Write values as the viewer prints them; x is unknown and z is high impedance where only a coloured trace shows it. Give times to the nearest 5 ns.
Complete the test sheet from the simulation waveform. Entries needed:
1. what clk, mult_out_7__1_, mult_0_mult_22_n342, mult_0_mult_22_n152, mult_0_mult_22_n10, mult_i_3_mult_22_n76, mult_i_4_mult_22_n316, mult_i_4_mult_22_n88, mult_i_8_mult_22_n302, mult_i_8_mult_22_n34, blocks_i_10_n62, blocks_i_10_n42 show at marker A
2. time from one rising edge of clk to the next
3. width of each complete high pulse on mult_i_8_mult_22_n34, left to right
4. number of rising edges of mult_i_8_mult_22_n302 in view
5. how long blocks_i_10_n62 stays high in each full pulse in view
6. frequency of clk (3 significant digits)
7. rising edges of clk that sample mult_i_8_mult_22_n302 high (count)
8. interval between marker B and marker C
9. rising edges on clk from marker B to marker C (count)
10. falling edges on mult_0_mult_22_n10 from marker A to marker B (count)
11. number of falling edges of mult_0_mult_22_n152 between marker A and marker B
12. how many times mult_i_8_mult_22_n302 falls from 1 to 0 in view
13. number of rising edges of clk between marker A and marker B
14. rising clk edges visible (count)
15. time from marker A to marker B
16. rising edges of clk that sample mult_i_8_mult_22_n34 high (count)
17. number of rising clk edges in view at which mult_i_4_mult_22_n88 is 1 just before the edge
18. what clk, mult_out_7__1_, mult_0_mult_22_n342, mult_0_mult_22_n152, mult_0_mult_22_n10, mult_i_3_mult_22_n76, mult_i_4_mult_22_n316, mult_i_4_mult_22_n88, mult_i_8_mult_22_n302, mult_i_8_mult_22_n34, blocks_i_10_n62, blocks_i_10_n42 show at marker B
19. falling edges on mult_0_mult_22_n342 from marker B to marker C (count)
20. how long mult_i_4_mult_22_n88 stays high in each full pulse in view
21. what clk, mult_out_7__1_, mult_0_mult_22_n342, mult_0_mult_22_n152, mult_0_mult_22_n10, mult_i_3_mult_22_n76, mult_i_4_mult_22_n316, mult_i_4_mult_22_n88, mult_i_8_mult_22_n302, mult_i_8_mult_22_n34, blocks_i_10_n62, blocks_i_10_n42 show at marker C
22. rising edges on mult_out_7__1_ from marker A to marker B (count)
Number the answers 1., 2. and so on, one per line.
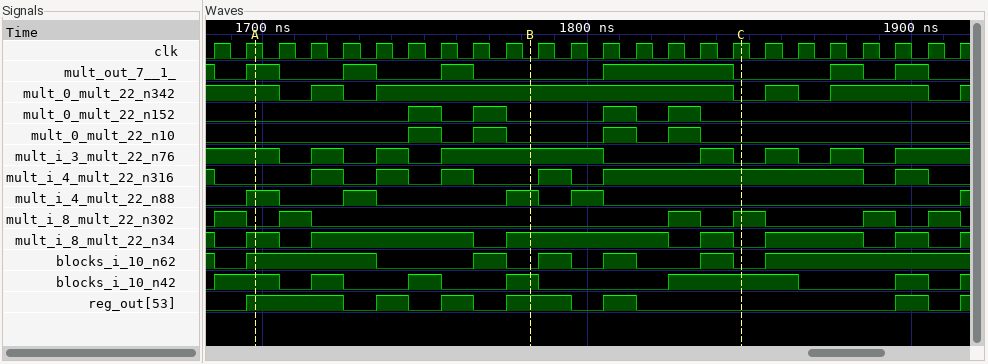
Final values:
1. clk=1, mult_out_7__1_=1, mult_0_mult_22_n342=1, mult_0_mult_22_n152=0, mult_0_mult_22_n10=0, mult_i_3_mult_22_n76=1, mult_i_4_mult_22_n316=0, mult_i_4_mult_22_n88=1, mult_i_8_mult_22_n302=0, mult_i_8_mult_22_n34=1, blocks_i_10_n62=1, blocks_i_10_n42=1
2. 10 ns
3. 10 ns, 50 ns, 50 ns, 10 ns, 30 ns, 10 ns
4. 6
5. 40 ns, 10 ns, 10 ns, 10 ns, 10 ns
6. 100 MHz
7. 6
8. 65 ns
9. 7
10. 2
11. 2
12. 6
13. 8
14. 24
15. 85 ns
16. 17
17. 4
18. clk=0, mult_out_7__1_=0, mult_0_mult_22_n342=1, mult_0_mult_22_n152=0, mult_0_mult_22_n10=0, mult_i_3_mult_22_n76=1, mult_i_4_mult_22_n316=0, mult_i_4_mult_22_n88=1, mult_i_8_mult_22_n302=0, mult_i_8_mult_22_n34=1, blocks_i_10_n62=0, blocks_i_10_n42=1
19. 1
20. 10 ns, 10 ns, 10 ns, 10 ns
21. clk=1, mult_out_7__1_=0, mult_0_mult_22_n342=0, mult_0_mult_22_n152=0, mult_0_mult_22_n10=0, mult_i_3_mult_22_n76=0, mult_i_4_mult_22_n316=1, mult_i_4_mult_22_n88=0, mult_i_8_mult_22_n302=1, mult_i_8_mult_22_n34=0, blocks_i_10_n62=0, blocks_i_10_n42=1
22. 2
